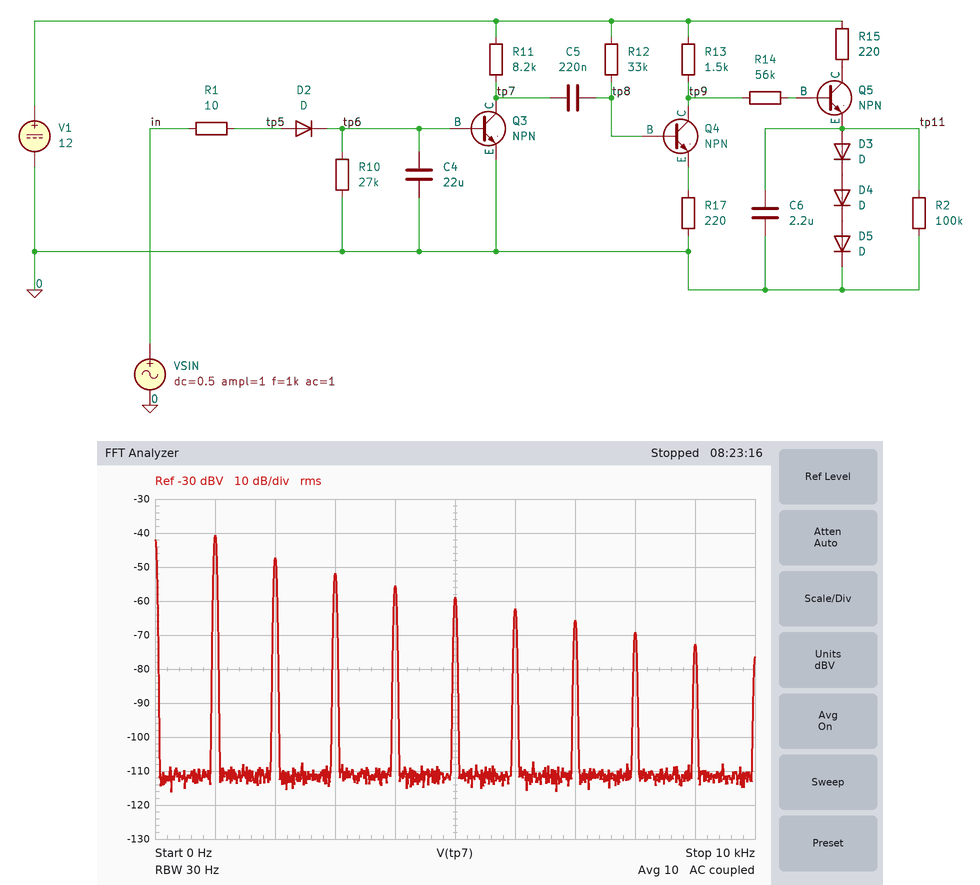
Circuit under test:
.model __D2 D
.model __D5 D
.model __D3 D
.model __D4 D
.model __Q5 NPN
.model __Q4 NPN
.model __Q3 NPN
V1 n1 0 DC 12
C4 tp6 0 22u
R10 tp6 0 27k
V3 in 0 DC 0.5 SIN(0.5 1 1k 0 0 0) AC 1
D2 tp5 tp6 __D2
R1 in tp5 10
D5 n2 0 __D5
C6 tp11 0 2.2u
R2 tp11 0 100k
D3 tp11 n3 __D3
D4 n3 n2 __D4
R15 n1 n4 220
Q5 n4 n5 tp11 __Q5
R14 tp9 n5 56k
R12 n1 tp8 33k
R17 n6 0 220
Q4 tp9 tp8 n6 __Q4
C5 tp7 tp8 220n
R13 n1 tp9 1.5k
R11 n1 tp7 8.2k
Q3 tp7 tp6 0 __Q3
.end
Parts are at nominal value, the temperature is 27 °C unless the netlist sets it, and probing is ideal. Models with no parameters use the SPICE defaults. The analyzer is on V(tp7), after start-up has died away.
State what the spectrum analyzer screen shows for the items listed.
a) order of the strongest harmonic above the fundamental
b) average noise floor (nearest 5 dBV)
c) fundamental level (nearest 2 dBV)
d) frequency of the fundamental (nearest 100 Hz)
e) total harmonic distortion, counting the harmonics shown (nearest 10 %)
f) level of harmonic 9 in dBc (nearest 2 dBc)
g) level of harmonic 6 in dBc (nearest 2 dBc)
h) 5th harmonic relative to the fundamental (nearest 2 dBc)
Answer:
2
-110 dBV
-40 dBV
1.0 kHz
60 %
-32 dBc
-22 dBc
-18 dBc
